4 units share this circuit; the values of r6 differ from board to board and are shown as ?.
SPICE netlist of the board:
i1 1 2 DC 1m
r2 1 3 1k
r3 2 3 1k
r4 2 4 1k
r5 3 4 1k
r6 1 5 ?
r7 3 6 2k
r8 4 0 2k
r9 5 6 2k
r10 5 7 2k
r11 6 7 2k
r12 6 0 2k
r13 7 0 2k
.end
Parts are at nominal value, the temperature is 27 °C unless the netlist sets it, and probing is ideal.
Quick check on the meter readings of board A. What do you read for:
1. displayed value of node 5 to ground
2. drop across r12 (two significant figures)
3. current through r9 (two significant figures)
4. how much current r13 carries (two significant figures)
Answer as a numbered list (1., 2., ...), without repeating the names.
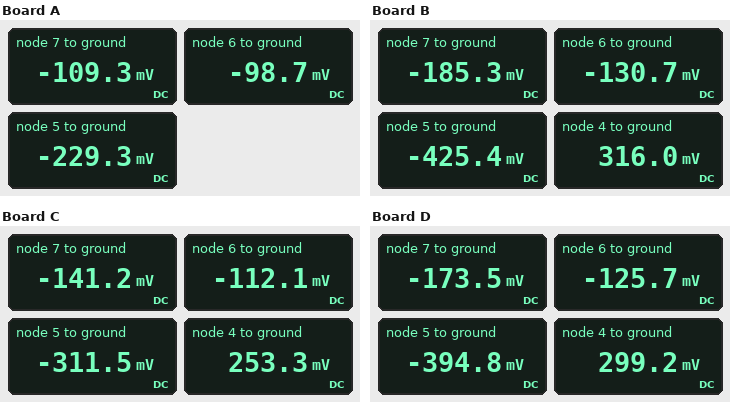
1. -229.3 mV
2. 99 mV
3. 65 µA
4. 55 µA
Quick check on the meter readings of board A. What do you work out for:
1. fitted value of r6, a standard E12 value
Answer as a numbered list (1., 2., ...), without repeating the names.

1. 5.6 kΩ
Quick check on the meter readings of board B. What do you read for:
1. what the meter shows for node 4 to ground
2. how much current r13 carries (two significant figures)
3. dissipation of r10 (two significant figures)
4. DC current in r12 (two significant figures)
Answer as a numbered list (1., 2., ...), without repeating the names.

1. 316.0 mV
2. 93 µA
3. 29 µW
4. 65 µA
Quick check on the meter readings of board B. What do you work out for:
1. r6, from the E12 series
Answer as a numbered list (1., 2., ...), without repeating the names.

1. 820 Ω
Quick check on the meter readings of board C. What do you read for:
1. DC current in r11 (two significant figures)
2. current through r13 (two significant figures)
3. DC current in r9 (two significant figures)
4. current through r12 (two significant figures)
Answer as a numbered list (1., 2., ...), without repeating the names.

1. 15 µA
2. 71 µA
3. 100 µA
4. 56 µA
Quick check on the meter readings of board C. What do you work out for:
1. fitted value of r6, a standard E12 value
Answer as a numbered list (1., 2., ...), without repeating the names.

1. 2.7 kΩ
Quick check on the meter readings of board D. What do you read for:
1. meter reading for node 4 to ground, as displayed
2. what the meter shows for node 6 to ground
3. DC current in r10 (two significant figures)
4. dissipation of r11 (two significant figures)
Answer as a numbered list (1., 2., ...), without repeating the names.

1. 299.2 mV
2. -125.7 mV
3. 110 µA
4. 1.1 µW
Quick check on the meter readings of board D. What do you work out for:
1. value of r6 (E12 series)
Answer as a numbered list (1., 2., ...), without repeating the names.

1. 1.2 kΩ
